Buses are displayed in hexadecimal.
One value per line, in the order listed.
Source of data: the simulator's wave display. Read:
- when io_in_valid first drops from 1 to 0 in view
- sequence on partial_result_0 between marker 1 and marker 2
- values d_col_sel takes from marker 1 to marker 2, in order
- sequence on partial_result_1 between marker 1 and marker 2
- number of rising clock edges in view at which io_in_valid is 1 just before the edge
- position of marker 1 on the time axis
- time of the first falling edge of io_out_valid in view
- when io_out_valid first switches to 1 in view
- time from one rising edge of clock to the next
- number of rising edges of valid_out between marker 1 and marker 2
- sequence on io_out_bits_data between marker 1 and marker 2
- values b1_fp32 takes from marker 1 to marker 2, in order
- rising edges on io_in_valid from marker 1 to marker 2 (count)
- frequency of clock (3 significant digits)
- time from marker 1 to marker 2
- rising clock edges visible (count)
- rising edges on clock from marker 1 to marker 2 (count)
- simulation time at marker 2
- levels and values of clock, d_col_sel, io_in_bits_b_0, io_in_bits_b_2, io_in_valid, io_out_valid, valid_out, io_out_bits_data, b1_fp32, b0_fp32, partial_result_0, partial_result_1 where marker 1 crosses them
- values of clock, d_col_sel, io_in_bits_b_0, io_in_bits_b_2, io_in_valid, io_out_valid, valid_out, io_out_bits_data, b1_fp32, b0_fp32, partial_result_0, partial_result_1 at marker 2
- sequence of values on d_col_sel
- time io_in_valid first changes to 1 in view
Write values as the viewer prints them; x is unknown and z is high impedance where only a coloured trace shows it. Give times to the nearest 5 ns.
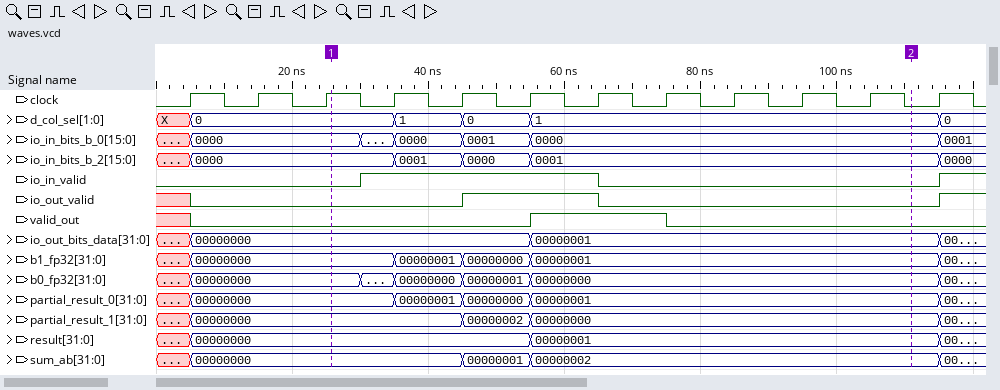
65 ns
00000000, 00000001, 00000000, 00000001
0, 1, 0, 1
00000000, 00000002, 00000000
4
25 ns
65 ns
45 ns
10 ns
1
00000000, 00000001
00000000, 00000001, 00000000, 00000001
1
100 MHz
85 ns
12
8
110 ns
clock=1, d_col_sel=0, io_in_bits_b_0=0000, io_in_bits_b_2=0000, io_in_valid=0, io_out_valid=0, valid_out=0, io_out_bits_data=00000000, b1_fp32=00000000, b0_fp32=00000000, partial_result_0=00000000, partial_result_1=00000000
clock=0, d_col_sel=1, io_in_bits_b_0=0000, io_in_bits_b_2=0001, io_in_valid=0, io_out_valid=0, valid_out=0, io_out_bits_data=00000001, b1_fp32=00000001, b0_fp32=00000000, partial_result_0=00000001, partial_result_1=00000000
X, 0, 1, 0, 1, 0
30 ns
